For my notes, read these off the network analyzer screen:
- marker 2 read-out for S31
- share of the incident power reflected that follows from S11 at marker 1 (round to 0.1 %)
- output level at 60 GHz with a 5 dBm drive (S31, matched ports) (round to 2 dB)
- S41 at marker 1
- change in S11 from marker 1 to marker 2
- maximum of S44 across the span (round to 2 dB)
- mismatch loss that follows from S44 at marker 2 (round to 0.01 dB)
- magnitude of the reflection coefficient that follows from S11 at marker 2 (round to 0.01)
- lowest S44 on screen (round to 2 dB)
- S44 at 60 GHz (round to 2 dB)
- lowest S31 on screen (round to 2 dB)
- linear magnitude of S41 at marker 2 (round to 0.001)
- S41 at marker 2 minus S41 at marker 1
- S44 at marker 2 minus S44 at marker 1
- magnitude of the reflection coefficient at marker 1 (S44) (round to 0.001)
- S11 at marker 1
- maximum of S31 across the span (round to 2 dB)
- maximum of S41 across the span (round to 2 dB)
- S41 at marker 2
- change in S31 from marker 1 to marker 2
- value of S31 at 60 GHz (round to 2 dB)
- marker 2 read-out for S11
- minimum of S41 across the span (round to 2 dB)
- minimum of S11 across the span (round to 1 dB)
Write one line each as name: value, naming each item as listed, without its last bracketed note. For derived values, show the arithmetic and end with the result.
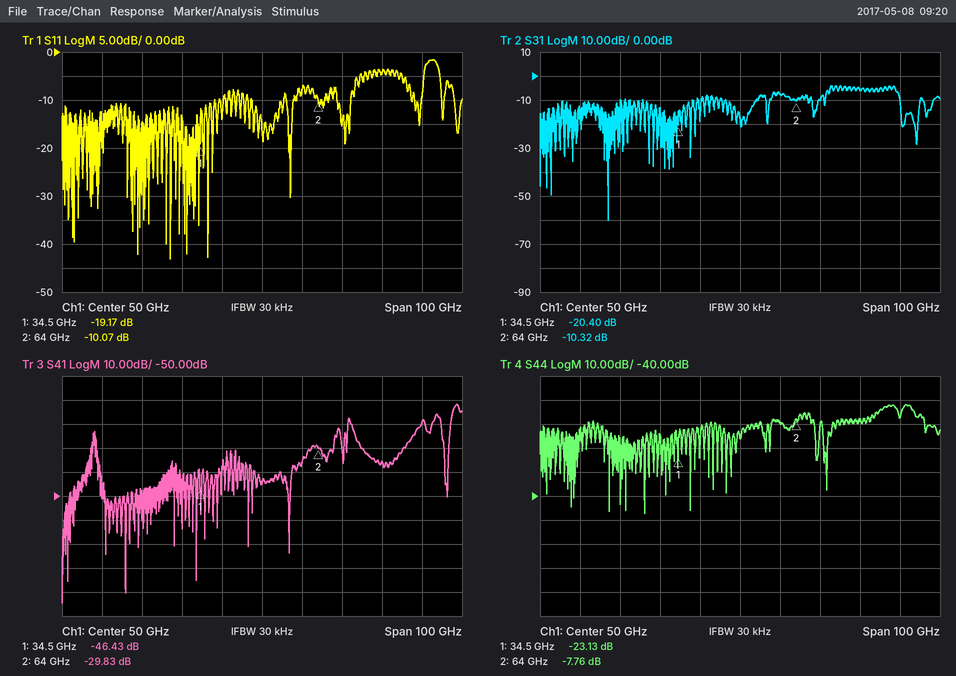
marker 2 read-out for S31: -10.32 dB
share of the incident power reflected that follows from S11 at marker 1: 10^(-19.17/10) ≈ 1.2 %
output level at 60 GHz with a 5 dBm drive (S31, matched ports): 5 dBm + (-8 dB) = -2 dBm
S41 at marker 1: -46.43 dB
change in S11 from marker 1 to marker 2: -10.07 − (-19.17) = 9.10 dB
maximum of S44 across the span: -2 dB
mismatch loss that follows from S44 at marker 2: −10 log10(1 − 10^(-7.76/10)) ≈ 0.80 dB
magnitude of the reflection coefficient that follows from S11 at marker 2: 10^(-10.07/20) ≈ 0.31
lowest S44 on screen: -48 dB
S44 at 60 GHz: -10 dB
lowest S31 on screen: -60 dB
linear magnitude of S41 at marker 2: 10^(-29.83/20) ≈ 0.032
S41 at marker 2 minus S41 at marker 1: -29.83 − (-46.43) = 16.60 dB
S44 at marker 2 minus S44 at marker 1: -7.76 − (-23.13) = 15.37 dB
magnitude of the reflection coefficient at marker 1 (S44): 10^(-23.13/20) ≈ 0.070
S11 at marker 1: -19.17 dB
maximum of S31 across the span: -4 dB
maximum of S41 across the span: -12 dB
S41 at marker 2: -29.83 dB
change in S31 from marker 1 to marker 2: -10.32 − (-20.4) = 10.08 dB
value of S31 at 60 GHz: -8 dB
marker 2 read-out for S11: -10.07 dB
minimum of S41 across the span: -94 dB
minimum of S11 across the span: -43 dB
